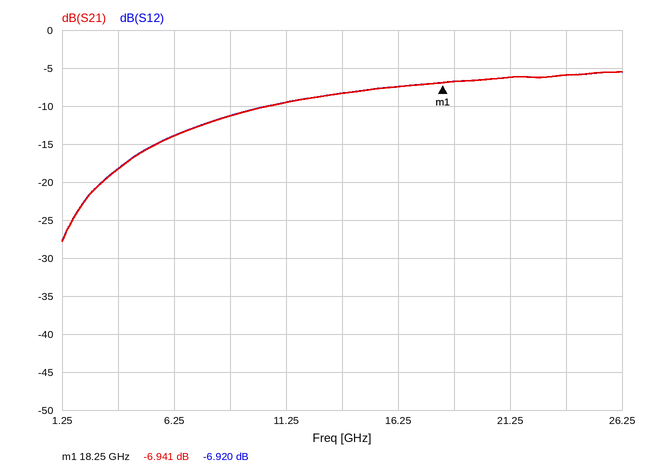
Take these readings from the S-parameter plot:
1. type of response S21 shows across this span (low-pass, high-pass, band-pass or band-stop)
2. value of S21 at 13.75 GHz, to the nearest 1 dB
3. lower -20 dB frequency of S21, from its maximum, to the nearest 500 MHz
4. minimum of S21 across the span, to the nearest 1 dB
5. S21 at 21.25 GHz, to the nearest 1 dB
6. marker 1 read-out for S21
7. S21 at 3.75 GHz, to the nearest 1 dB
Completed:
high-pass
-8 dB
1.5 GHz
-28 dB
-6 dB
-6.941 dB
-18 dB
